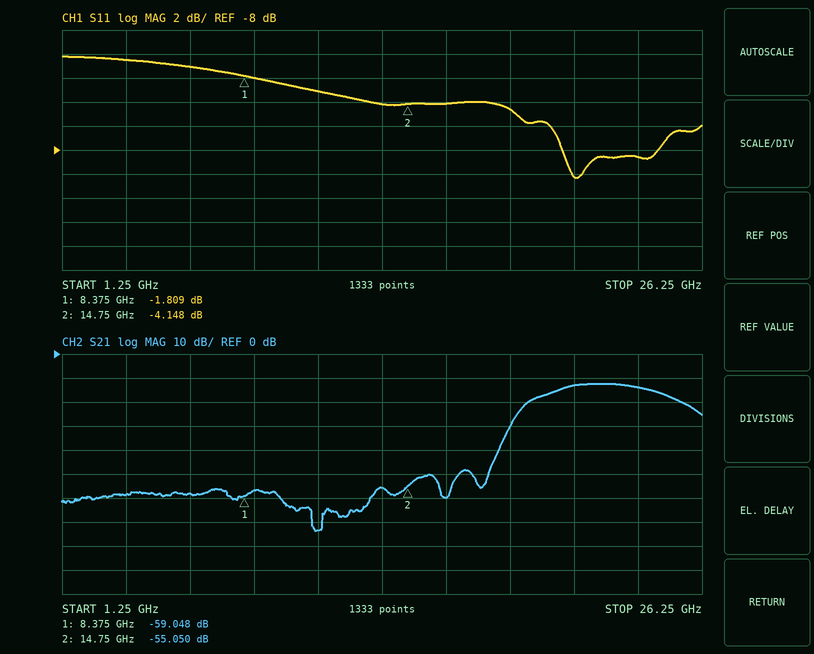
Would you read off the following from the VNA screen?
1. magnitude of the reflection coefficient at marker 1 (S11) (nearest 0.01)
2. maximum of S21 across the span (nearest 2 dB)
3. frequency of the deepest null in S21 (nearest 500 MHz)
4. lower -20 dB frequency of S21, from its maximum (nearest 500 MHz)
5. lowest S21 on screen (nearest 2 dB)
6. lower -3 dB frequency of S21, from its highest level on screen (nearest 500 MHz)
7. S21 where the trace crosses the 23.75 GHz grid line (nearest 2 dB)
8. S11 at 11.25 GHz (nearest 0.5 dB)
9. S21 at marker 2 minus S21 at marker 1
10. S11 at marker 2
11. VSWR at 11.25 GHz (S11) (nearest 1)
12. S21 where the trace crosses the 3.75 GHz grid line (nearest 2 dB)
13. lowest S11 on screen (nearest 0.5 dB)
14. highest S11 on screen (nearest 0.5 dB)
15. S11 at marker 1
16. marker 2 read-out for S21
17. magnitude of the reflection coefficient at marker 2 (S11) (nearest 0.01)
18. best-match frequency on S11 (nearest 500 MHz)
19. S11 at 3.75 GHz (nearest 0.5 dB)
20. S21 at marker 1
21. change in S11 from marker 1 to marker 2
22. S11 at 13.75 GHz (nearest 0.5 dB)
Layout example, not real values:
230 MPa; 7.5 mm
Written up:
0.81; -12 dB; 11.0 GHz; 18.5 GHz; -74 dB; 20.5 GHz; -14 dB; -3.0 dB; 3.998 dB; -4.148 dB; 6; -58 dB; -10.5 dB; 0.0 dB; -1.809 dB; -55.050 dB; 0.62; 21.5 GHz; -0.5 dB; -59.048 dB; -2.339 dB; -4.0 dB
